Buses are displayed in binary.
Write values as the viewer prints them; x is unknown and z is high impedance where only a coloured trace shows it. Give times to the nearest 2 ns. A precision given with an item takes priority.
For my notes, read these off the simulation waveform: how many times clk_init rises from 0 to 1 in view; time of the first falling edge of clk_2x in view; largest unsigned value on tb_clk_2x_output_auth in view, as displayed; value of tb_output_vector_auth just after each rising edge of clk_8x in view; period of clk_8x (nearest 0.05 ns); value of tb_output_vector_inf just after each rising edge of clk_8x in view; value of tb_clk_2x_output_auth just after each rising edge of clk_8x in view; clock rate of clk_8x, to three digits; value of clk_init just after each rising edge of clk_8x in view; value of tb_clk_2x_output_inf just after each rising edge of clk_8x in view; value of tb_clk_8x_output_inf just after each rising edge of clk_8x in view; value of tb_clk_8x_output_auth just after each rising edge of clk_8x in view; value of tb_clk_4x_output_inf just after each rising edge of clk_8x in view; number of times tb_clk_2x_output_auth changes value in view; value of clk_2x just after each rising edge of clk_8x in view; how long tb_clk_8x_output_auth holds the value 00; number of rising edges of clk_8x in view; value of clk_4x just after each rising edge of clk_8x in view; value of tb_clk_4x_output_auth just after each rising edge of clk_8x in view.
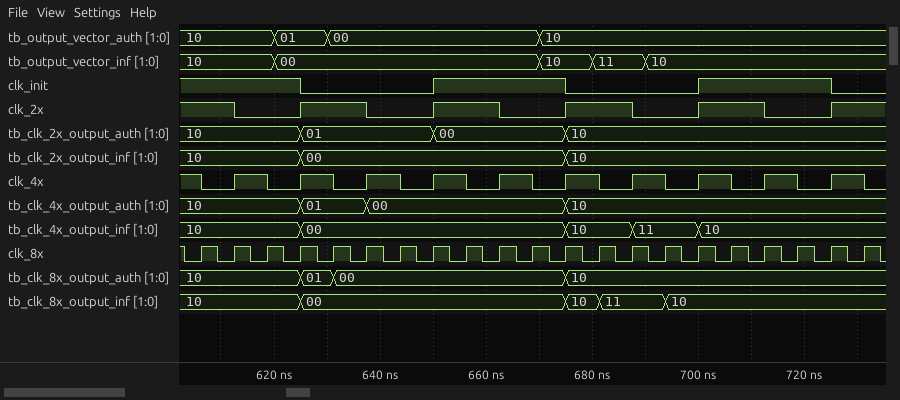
2
612 ns
10
10, 10, 10, 01, 00, 00, 00, 00, 00, 00, 00, 10, 10, 10, 10, 10, 10, 10, 10, 10, 10
6.25 ns
10, 10, 10, 00, 00, 00, 00, 00, 00, 00, 00, 10, 11, 11, 10, 10, 10, 10, 10, 10, 10
10, 10, 10, 01, 01, 01, 01, 00, 00, 00, 00, 10, 10, 10, 10, 10, 10, 10, 10, 10, 10
160 MHz
1 1 1 0 0 0 0 1 1 1 1 0 0 0 0 1 1 1 1 0 0
10, 10, 10, 00, 00, 00, 00, 00, 00, 00, 00, 10, 10, 10, 10, 10, 10, 10, 10, 10, 10
10, 10, 10, 00, 00, 00, 00, 00, 00, 00, 00, 10, 11, 11, 10, 10, 10, 10, 10, 10, 10
10, 10, 10, 01, 00, 00, 00, 00, 00, 00, 00, 10, 10, 10, 10, 10, 10, 10, 10, 10, 10
10, 10, 10, 00, 00, 00, 00, 00, 00, 00, 00, 10, 10, 11, 11, 10, 10, 10, 10, 10, 10
3
1 0 0 1 1 0 0 1 1 0 0 1 1 0 0 1 1 0 0 1 1
44 ns
21
0 1 0 1 0 1 0 1 0 1 0 1 0 1 0 1 0 1 0 1 0
10, 10, 10, 01, 01, 00, 00, 00, 00, 00, 00, 10, 10, 10, 10, 10, 10, 10, 10, 10, 10
